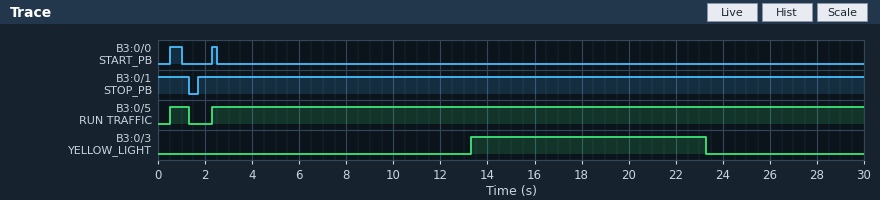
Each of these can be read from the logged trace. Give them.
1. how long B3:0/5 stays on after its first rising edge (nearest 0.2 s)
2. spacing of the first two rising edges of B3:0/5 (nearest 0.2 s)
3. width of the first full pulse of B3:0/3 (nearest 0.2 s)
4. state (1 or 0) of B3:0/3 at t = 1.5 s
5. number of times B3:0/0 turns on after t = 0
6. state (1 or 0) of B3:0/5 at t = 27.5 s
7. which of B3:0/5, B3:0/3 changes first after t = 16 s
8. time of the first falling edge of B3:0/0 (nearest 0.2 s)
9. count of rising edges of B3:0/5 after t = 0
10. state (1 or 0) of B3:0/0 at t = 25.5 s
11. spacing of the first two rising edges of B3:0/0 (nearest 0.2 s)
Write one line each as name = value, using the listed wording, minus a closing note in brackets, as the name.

how long B3:0/5 stays on after its first rising edge = 0.8 s
spacing of the first two rising edges of B3:0/5 = 1.8 s
width of the first full pulse of B3:0/3 = 10.0 s
state (1 or 0) of B3:0/3 at t = 1.5 s = 0
number of times B3:0/0 turns on after t = 0 = 2
state (1 or 0) of B3:0/5 at t = 27.5 s = 1
which of B3:0/5, B3:0/3 changes first after t = 16 s = B3:0/3
time of the first falling edge of B3:0/0 = 1.0 s
count of rising edges of B3:0/5 after t = 0 = 2
state (1 or 0) of B3:0/0 at t = 25.5 s = 0
spacing of the first two rising edges of B3:0/0 = 1.8 s
